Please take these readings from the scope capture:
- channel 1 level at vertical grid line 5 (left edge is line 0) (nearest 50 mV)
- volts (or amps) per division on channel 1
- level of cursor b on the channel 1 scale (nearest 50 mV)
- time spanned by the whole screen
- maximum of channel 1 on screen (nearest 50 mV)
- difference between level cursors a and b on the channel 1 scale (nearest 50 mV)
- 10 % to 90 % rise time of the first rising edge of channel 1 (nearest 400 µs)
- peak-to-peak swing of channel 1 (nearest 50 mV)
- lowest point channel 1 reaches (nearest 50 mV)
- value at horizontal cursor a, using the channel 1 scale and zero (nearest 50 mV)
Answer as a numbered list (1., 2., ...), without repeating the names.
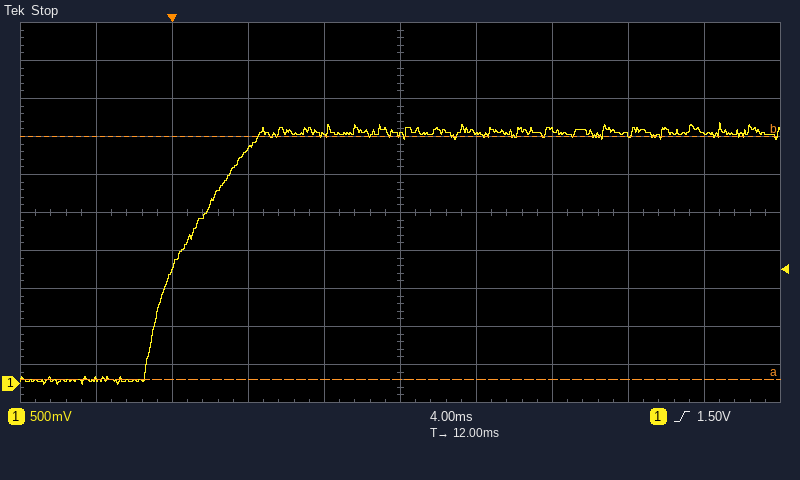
1. 3.25 V
2. 500 mV
3. 3.25 V
4. 40 ms
5. 3.45 V
6. 3.20 V
7. 4.8 ms
8. 3.45 V
9. 0 mV
10. 50 mV
